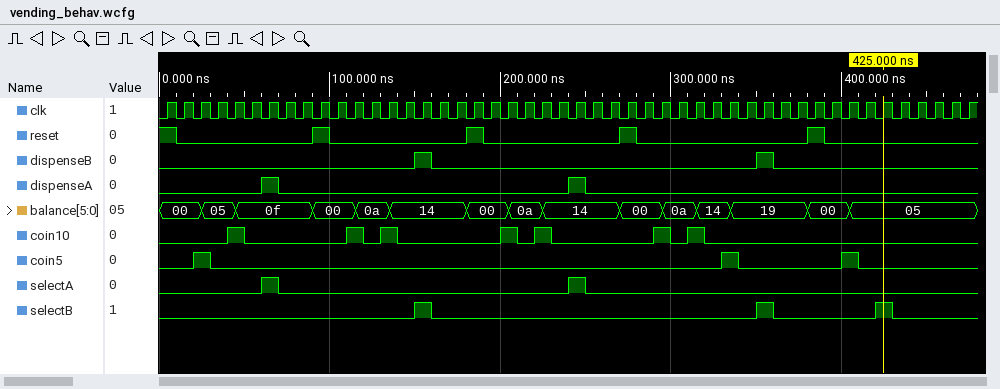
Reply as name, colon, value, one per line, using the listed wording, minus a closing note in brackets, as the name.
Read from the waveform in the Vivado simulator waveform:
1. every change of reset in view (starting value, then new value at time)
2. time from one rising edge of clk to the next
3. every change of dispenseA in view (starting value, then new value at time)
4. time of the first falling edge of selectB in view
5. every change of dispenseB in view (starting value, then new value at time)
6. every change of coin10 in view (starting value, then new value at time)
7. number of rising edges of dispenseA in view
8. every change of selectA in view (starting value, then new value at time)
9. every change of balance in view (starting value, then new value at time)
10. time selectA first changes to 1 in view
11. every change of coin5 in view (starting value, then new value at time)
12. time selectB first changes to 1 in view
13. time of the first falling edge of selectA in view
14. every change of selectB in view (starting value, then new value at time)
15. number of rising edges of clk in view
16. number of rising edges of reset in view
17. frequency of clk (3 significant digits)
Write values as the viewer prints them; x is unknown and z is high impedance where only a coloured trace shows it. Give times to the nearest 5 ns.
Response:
every change of reset in view: 1, 0 at 10 ns, 1 at 90 ns, 0 at 100 ns, 1 at 180 ns, 0 at 190 ns, 1 at 270 ns, 0 at 280 ns, 1 at 380 ns, 0 at 390 ns
time from one rising edge of clk to the next: 10 ns
every change of dispenseA in view: 0, 1 at 60 ns, 0 at 70 ns, 1 at 240 ns, 0 at 250 ns
time of the first falling edge of selectB in view: 160 ns
every change of dispenseB in view: 0, 1 at 150 ns, 0 at 160 ns, 1 at 350 ns, 0 at 360 ns
every change of coin10 in view: 0, 1 at 40 ns, 0 at 50 ns, 1 at 110 ns, 0 at 120 ns, 1 at 130 ns, 0 at 140 ns, 1 at 200 ns, 0 at 210 ns, 1 at 220 ns, 0 at 230 ns, 1 at 290 ns, 0 at 300 ns, 1 at 310 ns, 0 at 320 ns
number of rising edges of dispenseA in view: 2
every change of selectA in view: 0, 1 at 60 ns, 0 at 70 ns, 1 at 240 ns, 0 at 250 ns
every change of balance in view: 00, 05 at 25 ns, 0f at 45 ns, 00 at 90 ns, 0a at 115 ns, 14 at 135 ns, 00 at 180 ns, 0a at 205 ns, 14 at 225 ns, 00 at 270 ns, 0a at 295 ns, 14 at 315 ns, 19 at 335 ns, 00 at 380 ns, 05 at 405 ns
time selectA first changes to 1 in view: 60 ns
every change of coin5 in view: 0, 1 at 20 ns, 0 at 30 ns, 1 at 330 ns, 0 at 340 ns, 1 at 400 ns, 0 at 410 ns
time selectB first changes to 1 in view: 150 ns
time of the first falling edge of selectA in view: 70 ns
every change of selectB in view: 0, 1 at 150 ns, 0 at 160 ns, 1 at 350 ns, 0 at 360 ns, 1 at 420 ns, 0 at 430 ns
number of rising edges of clk in view: 48
number of rising edges of reset in view: 4
frequency of clk: 100 MHz
